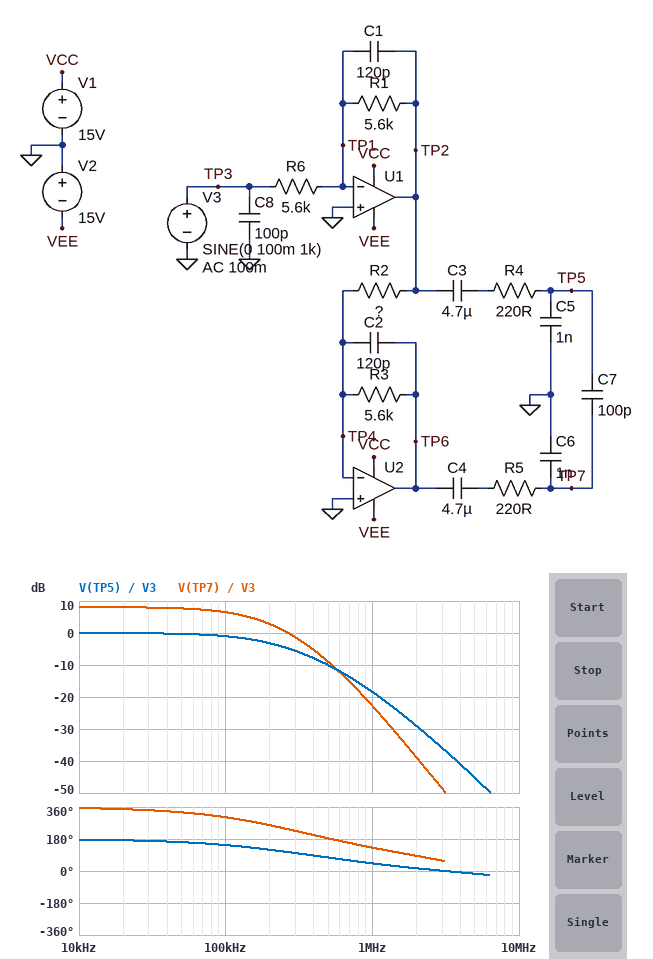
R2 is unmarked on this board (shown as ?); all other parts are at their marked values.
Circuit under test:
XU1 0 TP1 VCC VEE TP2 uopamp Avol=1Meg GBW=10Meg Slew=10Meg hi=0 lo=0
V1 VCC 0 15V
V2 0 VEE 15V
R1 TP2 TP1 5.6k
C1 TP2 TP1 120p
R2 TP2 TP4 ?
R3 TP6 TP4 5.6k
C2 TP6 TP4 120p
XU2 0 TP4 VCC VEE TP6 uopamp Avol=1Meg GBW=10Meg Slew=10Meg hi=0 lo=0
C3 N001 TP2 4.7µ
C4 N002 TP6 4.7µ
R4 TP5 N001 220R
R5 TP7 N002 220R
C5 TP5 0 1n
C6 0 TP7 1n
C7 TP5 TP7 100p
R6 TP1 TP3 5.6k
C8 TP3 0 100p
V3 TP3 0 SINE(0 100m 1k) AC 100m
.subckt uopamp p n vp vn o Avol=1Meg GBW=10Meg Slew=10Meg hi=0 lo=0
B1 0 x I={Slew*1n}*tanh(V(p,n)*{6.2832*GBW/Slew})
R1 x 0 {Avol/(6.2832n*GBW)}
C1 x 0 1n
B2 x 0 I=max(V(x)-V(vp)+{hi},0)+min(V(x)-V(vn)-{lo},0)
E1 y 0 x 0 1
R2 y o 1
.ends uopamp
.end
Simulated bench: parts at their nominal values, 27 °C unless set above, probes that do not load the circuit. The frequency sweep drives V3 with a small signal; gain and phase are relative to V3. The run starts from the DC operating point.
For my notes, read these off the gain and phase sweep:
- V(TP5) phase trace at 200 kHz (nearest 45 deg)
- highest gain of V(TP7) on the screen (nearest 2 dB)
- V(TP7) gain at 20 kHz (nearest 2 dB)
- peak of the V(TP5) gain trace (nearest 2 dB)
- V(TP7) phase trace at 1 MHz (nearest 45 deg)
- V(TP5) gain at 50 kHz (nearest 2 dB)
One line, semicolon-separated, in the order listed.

135 deg; 8 dB; 8 dB; 0 dB; 135 deg; 0 dB
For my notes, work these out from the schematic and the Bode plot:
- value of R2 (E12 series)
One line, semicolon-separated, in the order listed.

2.2 kΩ
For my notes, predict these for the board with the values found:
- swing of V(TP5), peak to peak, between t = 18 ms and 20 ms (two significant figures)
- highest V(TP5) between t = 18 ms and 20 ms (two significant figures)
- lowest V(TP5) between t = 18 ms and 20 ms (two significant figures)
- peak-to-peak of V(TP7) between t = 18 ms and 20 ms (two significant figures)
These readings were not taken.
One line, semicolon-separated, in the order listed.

200 mV; 100 mV; -100 mV; 510 mV
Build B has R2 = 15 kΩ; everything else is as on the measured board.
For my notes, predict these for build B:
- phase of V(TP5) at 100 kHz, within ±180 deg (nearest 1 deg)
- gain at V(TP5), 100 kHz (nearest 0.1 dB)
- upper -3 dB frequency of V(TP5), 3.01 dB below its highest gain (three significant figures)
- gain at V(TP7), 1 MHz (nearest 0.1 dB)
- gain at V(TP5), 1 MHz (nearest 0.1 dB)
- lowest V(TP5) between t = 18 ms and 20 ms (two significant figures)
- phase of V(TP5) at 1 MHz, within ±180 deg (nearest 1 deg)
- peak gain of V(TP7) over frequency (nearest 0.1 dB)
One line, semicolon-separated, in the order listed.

147 deg; -0.9 dB; 206 kHz; -35.5 dB; -18.2 dB; -100 mV; 41 deg; -8.6 dB
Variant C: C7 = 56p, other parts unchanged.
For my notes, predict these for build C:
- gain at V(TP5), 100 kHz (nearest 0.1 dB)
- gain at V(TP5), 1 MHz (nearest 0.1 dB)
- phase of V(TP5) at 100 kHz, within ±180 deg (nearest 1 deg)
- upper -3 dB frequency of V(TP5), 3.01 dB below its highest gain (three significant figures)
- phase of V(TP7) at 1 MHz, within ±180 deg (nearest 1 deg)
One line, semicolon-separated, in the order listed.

-0.9 dB; -18.1 dB; 147 deg; 201 kHz; 135 deg
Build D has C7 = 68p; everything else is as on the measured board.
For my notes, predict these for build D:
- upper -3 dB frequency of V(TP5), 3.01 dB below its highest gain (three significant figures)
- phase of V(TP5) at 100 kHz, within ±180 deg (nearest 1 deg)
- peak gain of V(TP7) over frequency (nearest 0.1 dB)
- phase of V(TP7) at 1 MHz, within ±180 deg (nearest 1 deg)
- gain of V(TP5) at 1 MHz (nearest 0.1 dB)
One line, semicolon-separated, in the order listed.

198 kHz; 147 deg; 8.1 dB; 134 deg; -18.2 dB
